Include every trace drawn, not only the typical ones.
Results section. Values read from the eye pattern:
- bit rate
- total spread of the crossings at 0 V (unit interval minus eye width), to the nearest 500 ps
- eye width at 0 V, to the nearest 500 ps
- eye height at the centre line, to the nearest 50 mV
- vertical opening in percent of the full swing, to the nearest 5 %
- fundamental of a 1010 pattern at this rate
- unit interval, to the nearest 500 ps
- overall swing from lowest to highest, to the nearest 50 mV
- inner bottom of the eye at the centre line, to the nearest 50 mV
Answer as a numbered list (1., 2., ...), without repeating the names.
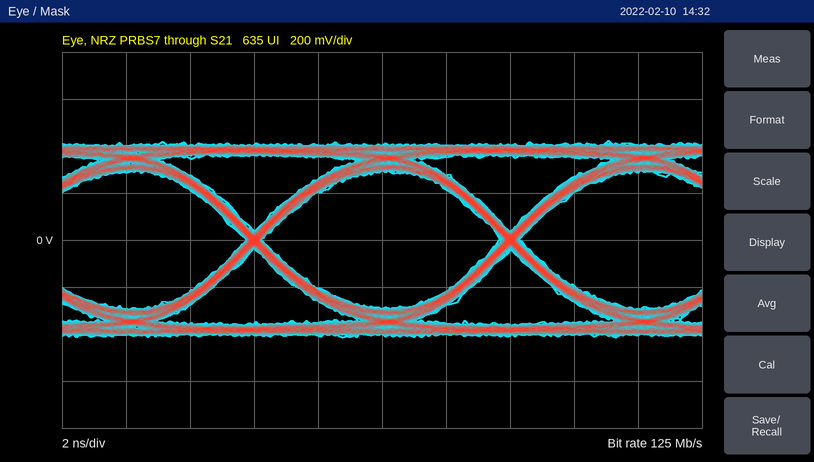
1. 125 Mb/s
2. 500 ps
3. 7.5 ns
4. 600 mV
5. 70 %
6. 62.5 MHz
7. 8.0 ns
8. 850 mV
9. -300 mV
